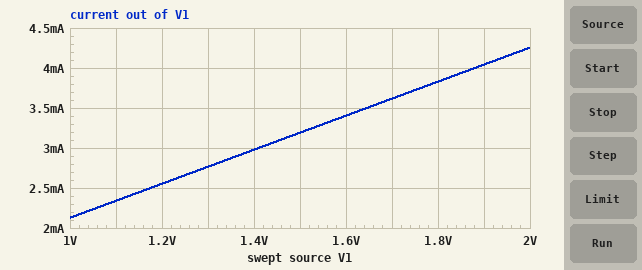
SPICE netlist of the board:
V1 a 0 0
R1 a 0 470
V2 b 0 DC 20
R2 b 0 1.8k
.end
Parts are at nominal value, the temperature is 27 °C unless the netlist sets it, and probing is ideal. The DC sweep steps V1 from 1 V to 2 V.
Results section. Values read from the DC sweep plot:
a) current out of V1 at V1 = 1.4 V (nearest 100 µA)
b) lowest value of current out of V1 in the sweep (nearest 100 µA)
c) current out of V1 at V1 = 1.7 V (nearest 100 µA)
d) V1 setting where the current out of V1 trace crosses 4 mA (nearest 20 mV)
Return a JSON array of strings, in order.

["3.0 mA", "2.1 mA", "3.6 mA", "1.88 V"]
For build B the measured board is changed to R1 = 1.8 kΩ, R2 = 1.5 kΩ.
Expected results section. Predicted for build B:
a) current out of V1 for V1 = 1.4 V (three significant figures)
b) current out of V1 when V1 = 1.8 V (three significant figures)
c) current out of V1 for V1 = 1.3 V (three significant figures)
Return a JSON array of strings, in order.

["778 µA", "1.00 mA", "722 µA"]
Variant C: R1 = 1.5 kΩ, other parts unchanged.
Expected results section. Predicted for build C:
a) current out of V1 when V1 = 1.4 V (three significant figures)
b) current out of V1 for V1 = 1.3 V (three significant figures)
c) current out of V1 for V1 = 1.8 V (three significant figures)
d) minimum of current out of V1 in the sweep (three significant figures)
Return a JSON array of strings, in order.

["933 µA", "867 µA", "1.20 mA", "667 µA"]
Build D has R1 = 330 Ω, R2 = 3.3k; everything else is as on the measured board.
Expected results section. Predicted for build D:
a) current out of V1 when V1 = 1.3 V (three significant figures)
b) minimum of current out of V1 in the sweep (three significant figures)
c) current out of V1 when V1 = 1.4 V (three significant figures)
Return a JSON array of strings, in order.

["3.94 mA", "3.03 mA", "4.24 mA"]
